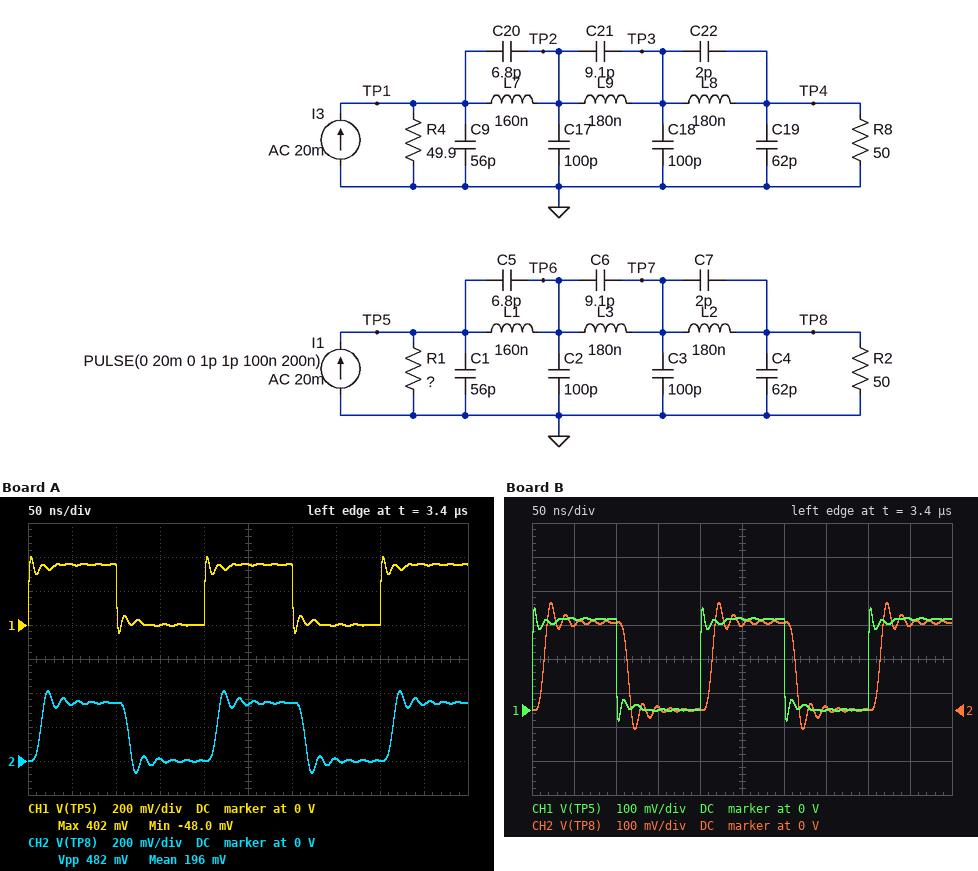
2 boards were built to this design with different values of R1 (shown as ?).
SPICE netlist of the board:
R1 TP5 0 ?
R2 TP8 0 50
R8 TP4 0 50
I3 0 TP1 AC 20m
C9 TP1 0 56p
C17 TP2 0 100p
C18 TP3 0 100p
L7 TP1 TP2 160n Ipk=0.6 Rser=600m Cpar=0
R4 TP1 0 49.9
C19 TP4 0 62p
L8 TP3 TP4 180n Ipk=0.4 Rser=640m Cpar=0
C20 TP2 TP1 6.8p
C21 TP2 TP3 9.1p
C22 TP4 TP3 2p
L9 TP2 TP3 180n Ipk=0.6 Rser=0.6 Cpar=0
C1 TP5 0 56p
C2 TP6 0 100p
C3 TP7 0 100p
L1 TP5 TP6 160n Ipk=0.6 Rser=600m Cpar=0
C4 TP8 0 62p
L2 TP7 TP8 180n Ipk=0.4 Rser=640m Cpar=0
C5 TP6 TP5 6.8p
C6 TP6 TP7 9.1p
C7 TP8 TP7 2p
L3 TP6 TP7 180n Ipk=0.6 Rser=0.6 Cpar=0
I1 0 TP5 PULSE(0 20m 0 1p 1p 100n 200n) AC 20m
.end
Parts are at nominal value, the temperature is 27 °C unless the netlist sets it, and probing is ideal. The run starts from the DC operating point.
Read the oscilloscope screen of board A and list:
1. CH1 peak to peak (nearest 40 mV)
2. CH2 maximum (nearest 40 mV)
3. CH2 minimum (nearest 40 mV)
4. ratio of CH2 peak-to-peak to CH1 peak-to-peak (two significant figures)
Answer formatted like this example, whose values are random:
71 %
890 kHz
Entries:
440 mV
400 mV
-80 mV
1.1
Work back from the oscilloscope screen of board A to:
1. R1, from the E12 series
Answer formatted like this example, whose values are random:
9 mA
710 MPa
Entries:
27 Ω
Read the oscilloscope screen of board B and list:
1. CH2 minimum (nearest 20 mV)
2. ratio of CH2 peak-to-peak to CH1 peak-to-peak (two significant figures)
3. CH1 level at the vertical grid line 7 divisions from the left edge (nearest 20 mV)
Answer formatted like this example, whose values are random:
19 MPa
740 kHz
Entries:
-60 mV
1.1
0 V
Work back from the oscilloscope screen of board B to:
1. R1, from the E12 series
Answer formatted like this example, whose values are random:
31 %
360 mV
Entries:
18 Ω
